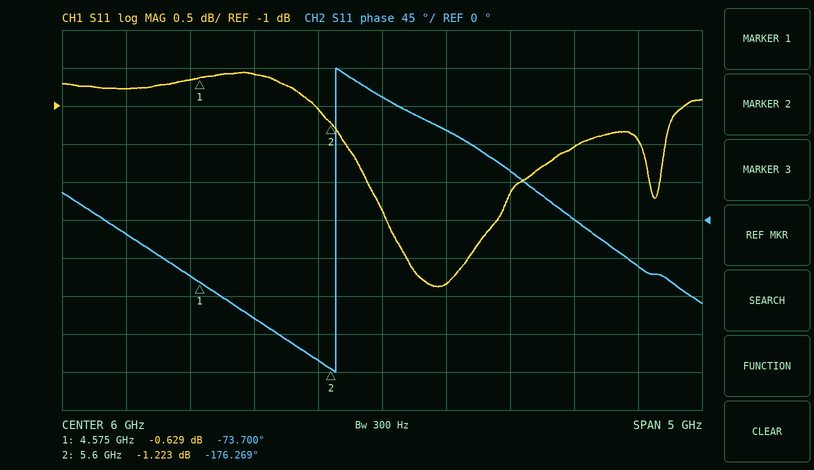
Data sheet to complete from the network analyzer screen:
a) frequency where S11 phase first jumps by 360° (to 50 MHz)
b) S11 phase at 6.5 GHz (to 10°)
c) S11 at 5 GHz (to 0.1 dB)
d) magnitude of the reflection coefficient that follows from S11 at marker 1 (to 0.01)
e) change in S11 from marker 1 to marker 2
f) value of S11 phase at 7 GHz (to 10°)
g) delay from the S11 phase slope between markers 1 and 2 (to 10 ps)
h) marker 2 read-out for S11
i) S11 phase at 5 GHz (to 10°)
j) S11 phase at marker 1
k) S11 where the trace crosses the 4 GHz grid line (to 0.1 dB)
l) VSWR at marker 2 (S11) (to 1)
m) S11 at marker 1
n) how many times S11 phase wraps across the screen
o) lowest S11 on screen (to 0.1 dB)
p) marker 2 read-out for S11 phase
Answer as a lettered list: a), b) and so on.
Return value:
a) 5.65 GHz
b) 110°
c) -0.6 dB
d) 0.93
e) -0.594 dB
f) 60°
g) 280 ps
h) -1.223 dB
i) -120°
j) -73.700°
k) -0.8 dB
l) 14
m) -0.629 dB
n) 1
o) -3.4 dB
p) -176.269°
